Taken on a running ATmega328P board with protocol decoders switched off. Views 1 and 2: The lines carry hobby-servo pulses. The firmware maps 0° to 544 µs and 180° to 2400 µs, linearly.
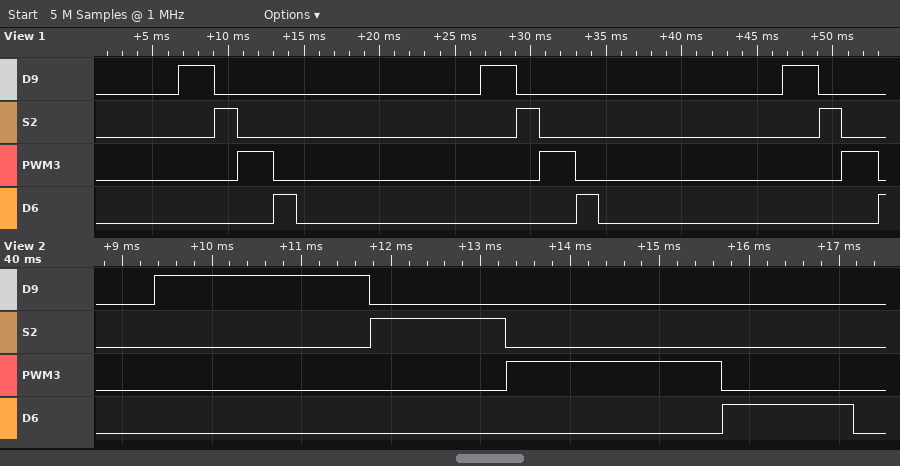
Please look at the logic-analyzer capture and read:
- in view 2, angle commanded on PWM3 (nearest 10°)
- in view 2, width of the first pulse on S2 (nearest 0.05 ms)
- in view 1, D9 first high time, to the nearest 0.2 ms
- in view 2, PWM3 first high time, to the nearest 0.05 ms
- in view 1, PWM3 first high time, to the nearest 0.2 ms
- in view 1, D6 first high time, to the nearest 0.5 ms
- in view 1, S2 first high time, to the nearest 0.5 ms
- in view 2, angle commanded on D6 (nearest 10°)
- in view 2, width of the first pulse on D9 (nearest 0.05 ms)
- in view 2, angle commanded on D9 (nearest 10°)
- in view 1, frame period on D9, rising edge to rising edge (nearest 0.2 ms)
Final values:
180°
1.50 ms
2.4 ms
2.40 ms
2.4 ms
1.5 ms
1.5 ms
90°
2.40 ms
180°
20.0 ms
